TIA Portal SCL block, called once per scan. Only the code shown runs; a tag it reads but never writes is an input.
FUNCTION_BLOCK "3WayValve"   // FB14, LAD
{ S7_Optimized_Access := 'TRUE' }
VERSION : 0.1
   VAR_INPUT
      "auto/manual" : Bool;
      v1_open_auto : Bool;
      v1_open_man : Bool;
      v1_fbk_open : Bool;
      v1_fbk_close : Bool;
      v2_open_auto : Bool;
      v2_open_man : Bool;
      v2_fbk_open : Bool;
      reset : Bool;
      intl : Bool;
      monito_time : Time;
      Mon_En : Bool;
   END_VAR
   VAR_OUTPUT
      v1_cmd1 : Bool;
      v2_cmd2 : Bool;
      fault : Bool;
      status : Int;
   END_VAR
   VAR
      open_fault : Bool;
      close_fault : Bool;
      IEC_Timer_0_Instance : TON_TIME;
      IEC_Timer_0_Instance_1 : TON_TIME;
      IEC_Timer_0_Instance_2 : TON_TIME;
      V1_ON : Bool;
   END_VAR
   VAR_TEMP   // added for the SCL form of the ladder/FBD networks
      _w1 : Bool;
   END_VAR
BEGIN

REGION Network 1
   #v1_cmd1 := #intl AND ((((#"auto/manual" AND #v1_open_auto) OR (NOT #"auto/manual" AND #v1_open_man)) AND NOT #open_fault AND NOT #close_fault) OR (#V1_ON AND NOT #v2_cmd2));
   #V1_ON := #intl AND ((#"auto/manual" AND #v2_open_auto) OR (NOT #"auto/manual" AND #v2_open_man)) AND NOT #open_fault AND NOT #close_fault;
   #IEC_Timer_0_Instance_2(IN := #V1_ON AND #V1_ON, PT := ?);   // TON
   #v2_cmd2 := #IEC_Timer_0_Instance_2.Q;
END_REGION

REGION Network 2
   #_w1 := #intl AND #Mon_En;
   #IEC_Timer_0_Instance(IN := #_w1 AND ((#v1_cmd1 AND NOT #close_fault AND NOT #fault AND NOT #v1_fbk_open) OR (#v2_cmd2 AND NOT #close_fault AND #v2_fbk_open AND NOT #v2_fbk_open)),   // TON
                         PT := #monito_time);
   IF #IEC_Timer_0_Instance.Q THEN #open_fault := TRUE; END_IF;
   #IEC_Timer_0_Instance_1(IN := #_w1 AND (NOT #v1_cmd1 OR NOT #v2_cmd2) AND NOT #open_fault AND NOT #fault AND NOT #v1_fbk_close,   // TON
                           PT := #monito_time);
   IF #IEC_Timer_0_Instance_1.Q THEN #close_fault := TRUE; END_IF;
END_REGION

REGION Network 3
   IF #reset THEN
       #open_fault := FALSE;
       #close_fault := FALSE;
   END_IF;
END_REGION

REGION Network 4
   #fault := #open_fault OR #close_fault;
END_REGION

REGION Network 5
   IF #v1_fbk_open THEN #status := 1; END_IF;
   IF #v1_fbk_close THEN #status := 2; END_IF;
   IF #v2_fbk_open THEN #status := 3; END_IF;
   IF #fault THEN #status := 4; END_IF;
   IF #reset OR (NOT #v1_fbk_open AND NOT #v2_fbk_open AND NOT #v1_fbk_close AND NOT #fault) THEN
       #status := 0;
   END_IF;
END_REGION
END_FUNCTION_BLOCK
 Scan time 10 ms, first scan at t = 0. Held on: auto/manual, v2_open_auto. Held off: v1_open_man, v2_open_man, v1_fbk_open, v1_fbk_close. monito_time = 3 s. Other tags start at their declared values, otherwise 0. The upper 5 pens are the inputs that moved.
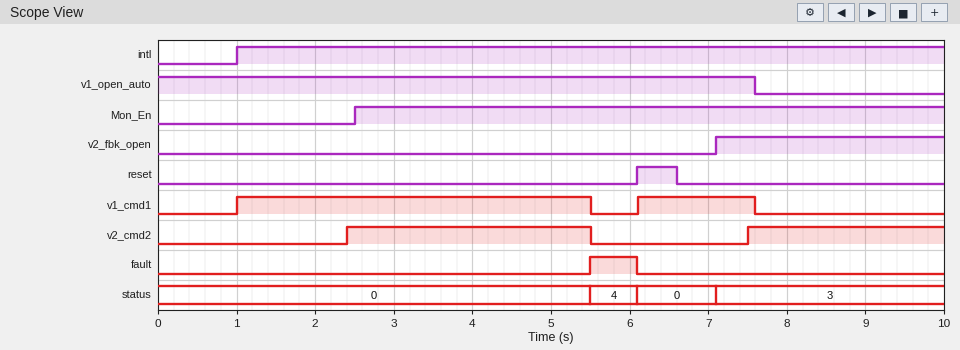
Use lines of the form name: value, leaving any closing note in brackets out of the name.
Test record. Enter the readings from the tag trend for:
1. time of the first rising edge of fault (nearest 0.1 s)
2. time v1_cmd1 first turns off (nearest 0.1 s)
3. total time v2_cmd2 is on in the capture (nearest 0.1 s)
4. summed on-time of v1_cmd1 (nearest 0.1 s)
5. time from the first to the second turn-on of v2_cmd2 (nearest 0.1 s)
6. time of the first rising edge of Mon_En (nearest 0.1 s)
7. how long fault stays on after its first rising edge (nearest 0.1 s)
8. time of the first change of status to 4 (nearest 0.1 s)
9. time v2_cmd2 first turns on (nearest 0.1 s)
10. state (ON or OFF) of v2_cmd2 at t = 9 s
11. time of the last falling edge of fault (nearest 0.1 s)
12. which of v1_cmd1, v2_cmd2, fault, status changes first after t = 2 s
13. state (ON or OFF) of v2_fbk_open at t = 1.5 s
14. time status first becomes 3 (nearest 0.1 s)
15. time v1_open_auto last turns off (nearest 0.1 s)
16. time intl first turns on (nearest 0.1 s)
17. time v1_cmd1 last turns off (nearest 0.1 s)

time of the first rising edge of fault: 5.5 s
time v1_cmd1 first turns off: 5.5 s
total time v2_cmd2 is on in the capture: 5.6 s
summed on-time of v1_cmd1: 6.0 s
time from the first to the second turn-on of v2_cmd2: 5.1 s
time of the first rising edge of Mon_En: 2.5 s
how long fault stays on after its first rising edge: 0.6 s
time of the first change of status to 4: 5.5 s
time v2_cmd2 first turns on: 2.4 s
state (ON or OFF) of v2_cmd2 at t = 9 s: ON
time of the last falling edge of fault: 6.1 s
which of v1_cmd1, v2_cmd2, fault, status changes first after t = 2 s: v2_cmd2
state (ON or OFF) of v2_fbk_open at t = 1.5 s: OFF
time status first becomes 3: 7.1 s
time v1_open_auto last turns off: 7.6 s
time intl first turns on: 1.0 s
time v1_cmd1 last turns off: 7.6 s
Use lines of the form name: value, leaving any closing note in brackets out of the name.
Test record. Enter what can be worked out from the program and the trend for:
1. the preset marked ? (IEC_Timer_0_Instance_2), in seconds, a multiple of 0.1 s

the preset marked ? (IEC_Timer_0_Instance_2), in seconds, a multiple of 0.1 s: 1.4 s
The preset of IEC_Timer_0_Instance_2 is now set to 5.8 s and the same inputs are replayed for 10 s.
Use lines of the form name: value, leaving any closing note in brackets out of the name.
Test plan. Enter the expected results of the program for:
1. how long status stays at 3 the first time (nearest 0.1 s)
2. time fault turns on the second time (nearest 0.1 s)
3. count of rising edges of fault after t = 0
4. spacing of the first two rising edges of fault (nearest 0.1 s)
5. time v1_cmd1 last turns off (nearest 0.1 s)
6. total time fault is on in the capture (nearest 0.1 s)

how long status stays at 3 the first time: 2.0 s
time fault turns on the second time: 9.1 s
count of rising edges of fault after t = 0: 2
spacing of the first two rising edges of fault: 3.6 s
time v1_cmd1 last turns off: 9.1 s
total time fault is on in the capture: 1.5 s
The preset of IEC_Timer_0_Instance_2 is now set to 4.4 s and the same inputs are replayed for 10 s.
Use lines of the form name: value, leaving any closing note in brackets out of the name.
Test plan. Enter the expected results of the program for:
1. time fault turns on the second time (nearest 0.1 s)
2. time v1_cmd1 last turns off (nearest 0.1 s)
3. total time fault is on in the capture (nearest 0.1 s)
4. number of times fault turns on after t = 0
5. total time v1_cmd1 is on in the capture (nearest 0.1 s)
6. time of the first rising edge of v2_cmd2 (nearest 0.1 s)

time fault turns on the second time: 9.1 s
time v1_cmd1 last turns off: 9.1 s
total time fault is on in the capture: 1.5 s
number of times fault turns on after t = 0: 2
total time v1_cmd1 is on in the capture: 7.5 s
time of the first rising edge of v2_cmd2: 5.4 s
